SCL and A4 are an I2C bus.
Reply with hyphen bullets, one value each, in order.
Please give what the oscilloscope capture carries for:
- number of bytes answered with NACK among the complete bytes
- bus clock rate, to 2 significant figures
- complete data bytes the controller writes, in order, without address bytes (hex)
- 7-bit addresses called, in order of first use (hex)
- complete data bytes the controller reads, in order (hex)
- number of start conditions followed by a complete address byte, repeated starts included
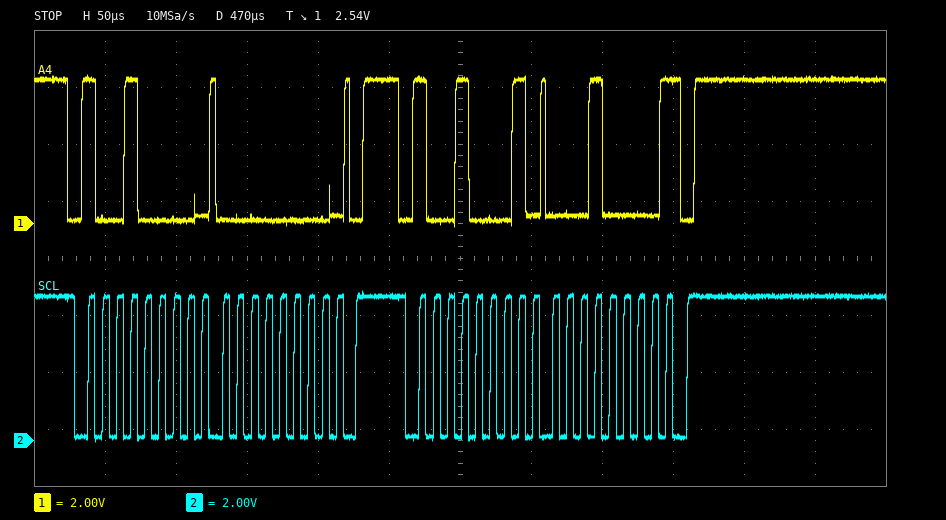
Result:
- 1
- 100 kHz
- 00
- 0x48
- 10
- 2
